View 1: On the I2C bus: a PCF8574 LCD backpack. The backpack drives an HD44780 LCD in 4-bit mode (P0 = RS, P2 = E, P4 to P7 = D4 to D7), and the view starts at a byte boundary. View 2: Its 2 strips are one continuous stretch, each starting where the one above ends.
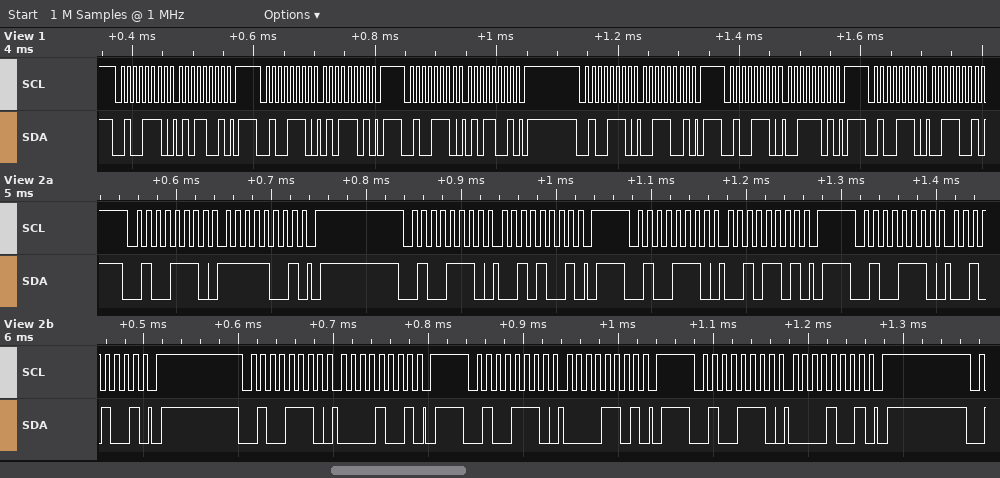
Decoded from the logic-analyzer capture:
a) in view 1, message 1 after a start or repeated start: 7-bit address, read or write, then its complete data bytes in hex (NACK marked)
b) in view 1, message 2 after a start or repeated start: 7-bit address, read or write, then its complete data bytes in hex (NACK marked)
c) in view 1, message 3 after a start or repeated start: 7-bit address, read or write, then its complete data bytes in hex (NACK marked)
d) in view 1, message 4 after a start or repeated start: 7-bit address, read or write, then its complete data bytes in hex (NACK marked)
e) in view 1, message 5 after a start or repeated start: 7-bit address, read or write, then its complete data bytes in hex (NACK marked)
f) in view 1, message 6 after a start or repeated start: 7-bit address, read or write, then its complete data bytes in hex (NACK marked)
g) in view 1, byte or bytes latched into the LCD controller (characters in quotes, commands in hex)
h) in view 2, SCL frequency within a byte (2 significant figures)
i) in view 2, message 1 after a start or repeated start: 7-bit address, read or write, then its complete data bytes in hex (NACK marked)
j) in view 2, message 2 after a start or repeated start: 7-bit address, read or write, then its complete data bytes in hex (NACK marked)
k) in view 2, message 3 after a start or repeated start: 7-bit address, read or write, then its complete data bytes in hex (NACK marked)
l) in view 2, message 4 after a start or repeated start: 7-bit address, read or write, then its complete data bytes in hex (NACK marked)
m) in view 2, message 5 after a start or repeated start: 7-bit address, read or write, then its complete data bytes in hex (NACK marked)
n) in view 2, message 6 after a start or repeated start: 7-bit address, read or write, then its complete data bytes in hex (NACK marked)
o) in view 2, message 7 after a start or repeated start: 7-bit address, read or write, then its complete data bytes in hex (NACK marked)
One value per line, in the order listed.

0x27 write: 59
0x27 write: 5D
0x27 write: 59
0x27 write: 39
0x27 write: 3D
0x27 write: 39
'S'
100 kHz
0x27 write: F9
0x27 write: 29
0x27 write: 2D
0x27 write: 29
0x27 write: 09
0x27 write: 0D
0x27 write: 09
